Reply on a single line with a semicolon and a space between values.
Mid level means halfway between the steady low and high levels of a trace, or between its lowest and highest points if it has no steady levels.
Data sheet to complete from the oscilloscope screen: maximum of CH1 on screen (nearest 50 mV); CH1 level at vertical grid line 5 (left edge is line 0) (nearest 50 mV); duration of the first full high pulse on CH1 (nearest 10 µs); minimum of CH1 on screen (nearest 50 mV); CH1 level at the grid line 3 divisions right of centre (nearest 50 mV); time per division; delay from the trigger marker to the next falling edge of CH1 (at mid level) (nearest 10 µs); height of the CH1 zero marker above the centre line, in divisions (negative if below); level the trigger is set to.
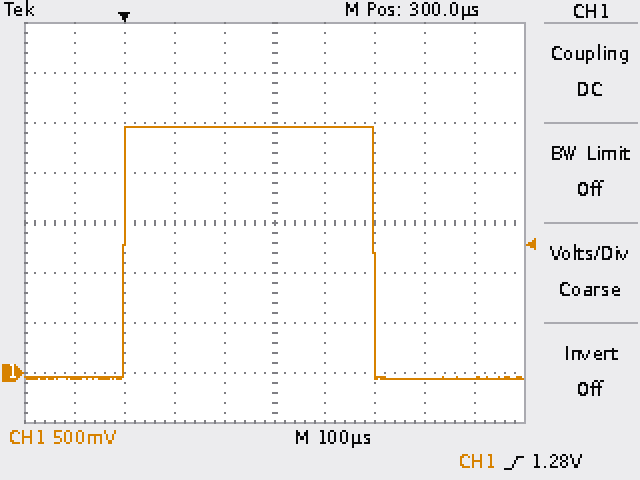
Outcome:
2.45 V; 2.45 V; 500 µs; -50 mV; -50 mV; 100 µs; 500 µs; -3.0 div; 1.28 V
